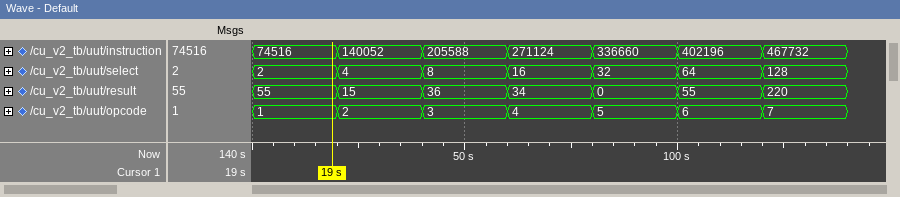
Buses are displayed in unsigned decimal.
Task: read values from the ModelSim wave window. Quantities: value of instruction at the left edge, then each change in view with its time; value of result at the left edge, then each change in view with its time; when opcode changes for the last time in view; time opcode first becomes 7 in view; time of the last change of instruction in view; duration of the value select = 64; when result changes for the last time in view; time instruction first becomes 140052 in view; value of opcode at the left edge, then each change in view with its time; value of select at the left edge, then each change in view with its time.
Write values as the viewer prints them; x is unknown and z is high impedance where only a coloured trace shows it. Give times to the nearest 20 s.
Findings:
74516, 140052 at 20 s, 205588 at 40 s, 271124 at 60 s, 336660 at 80 s, 402196 at 100 s, 467732 at 120 s
55, 15 at 20 s, 36 at 40 s, 34 at 60 s, 0 at 80 s, 55 at 100 s, 220 at 120 s
120 s
120 s
120 s
20 s
120 s
20 s
1, 2 at 20 s, 3 at 40 s, 4 at 60 s, 5 at 80 s, 6 at 100 s, 7 at 120 s
2, 4 at 20 s, 8 at 40 s, 16 at 60 s, 32 at 80 s, 64 at 100 s, 128 at 120 s
